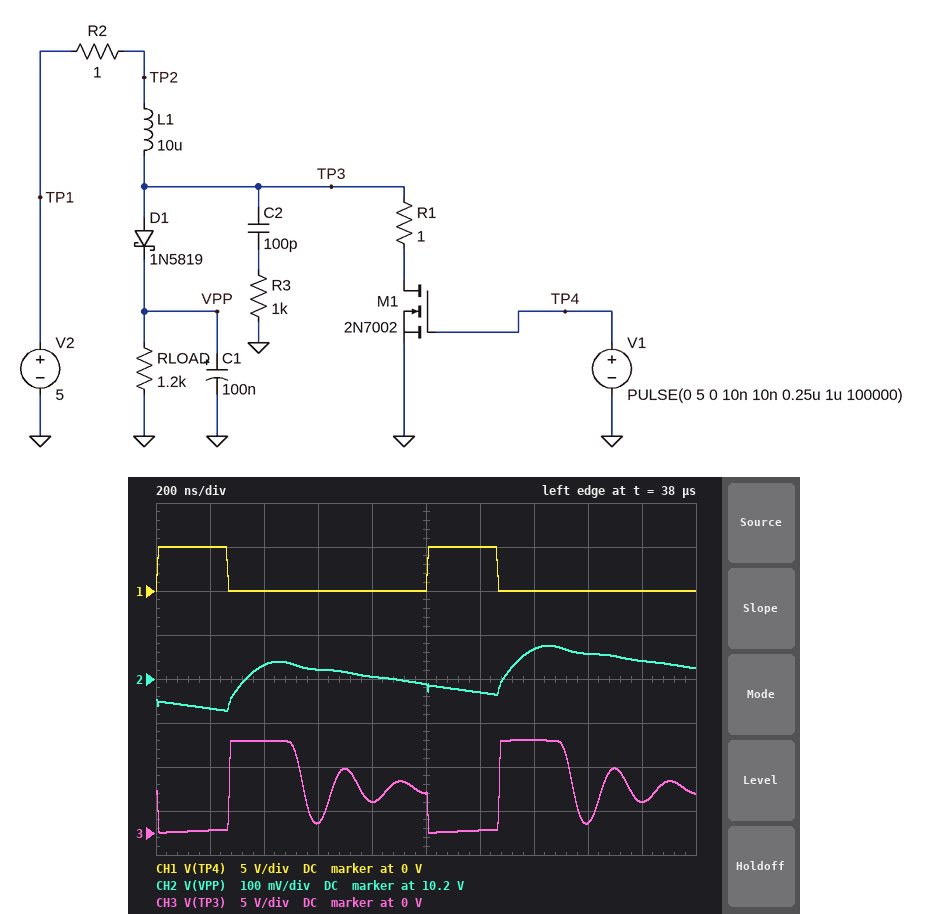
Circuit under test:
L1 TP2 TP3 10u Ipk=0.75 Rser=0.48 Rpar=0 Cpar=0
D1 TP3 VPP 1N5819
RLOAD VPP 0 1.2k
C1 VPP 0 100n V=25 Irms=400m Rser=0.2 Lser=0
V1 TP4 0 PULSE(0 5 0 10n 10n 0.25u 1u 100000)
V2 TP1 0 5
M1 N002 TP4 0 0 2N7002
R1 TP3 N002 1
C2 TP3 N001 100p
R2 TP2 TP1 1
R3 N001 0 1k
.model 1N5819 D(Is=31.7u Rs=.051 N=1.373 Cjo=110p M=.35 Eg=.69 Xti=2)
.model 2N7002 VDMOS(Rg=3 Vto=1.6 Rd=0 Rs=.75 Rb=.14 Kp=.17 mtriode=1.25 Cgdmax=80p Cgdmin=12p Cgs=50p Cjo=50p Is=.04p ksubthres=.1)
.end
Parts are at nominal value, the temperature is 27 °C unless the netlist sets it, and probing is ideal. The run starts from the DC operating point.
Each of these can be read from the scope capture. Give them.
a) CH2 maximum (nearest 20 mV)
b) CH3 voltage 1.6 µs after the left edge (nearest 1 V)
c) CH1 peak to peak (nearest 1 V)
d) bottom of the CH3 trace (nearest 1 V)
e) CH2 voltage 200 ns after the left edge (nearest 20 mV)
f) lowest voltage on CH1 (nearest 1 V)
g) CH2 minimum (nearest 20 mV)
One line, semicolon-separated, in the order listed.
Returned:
10.28 V; 1 V; 5 V; 0 V; 10.14 V; 0 V; 10.12 V
